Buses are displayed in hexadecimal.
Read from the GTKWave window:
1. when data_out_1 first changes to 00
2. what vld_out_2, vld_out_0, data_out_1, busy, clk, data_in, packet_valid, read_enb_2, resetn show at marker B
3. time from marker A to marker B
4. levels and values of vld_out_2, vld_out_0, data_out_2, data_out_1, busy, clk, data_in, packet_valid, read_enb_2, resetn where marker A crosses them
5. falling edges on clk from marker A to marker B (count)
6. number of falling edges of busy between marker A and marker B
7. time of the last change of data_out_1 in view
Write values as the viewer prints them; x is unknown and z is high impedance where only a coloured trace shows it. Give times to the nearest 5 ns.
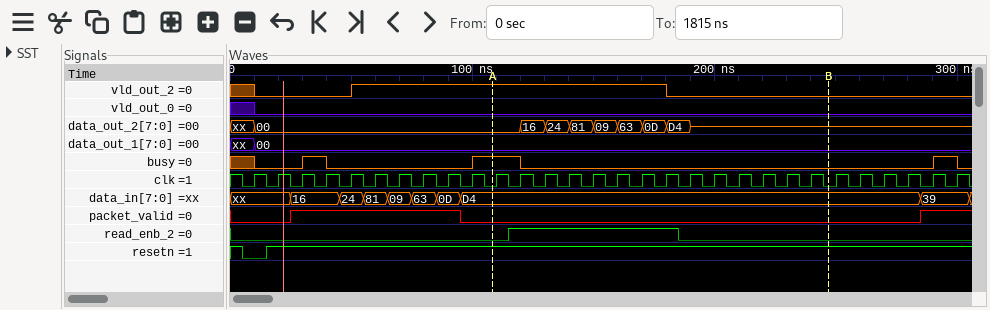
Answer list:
10 ns
vld_out_2=0, vld_out_0=0, data_out_1=00, busy=0, clk=0, data_in=D4, packet_valid=0, read_enb_2=0, resetn=1
140 ns
vld_out_2=1, vld_out_0=0, data_out_2=00, data_out_1=00, busy=1, clk=0, data_in=D4, packet_valid=0, read_enb_2=0, resetn=1
14
1
10 ns
